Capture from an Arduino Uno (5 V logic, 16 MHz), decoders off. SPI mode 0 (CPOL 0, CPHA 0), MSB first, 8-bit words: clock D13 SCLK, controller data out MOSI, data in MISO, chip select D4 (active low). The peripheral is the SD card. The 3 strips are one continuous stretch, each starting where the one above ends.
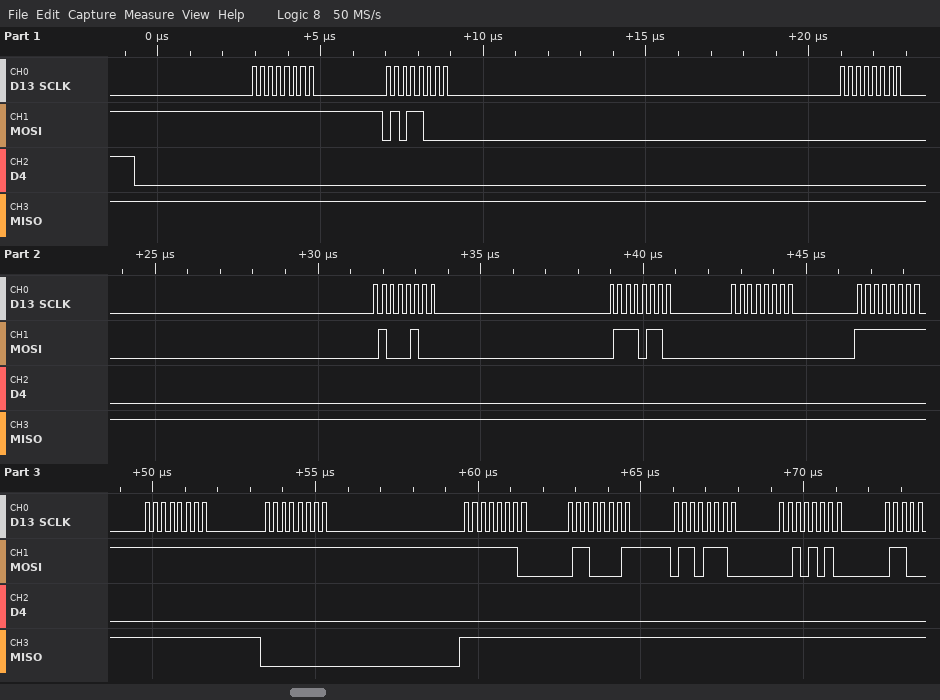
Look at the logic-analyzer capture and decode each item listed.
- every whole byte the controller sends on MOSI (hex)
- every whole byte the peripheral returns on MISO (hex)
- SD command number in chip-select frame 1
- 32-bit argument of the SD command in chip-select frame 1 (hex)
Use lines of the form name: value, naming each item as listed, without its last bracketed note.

every whole byte the controller sends on MOSI: 0xFF 0x58 0x00 0x44 0x76 0x00 0xFF 0xFF 0xFF 0xFE 0x61 0x6E 0x2A
every whole byte the peripheral returns on MISO: 0xFF 0xFF 0xFF 0xFF 0xFF 0xFF 0xFF 0xFF 0x00 0xFF 0xFF 0xFF 0xFF
SD command number in chip-select frame 1: CMD24
32-bit argument of the SD command in chip-select frame 1: 0x00447600
